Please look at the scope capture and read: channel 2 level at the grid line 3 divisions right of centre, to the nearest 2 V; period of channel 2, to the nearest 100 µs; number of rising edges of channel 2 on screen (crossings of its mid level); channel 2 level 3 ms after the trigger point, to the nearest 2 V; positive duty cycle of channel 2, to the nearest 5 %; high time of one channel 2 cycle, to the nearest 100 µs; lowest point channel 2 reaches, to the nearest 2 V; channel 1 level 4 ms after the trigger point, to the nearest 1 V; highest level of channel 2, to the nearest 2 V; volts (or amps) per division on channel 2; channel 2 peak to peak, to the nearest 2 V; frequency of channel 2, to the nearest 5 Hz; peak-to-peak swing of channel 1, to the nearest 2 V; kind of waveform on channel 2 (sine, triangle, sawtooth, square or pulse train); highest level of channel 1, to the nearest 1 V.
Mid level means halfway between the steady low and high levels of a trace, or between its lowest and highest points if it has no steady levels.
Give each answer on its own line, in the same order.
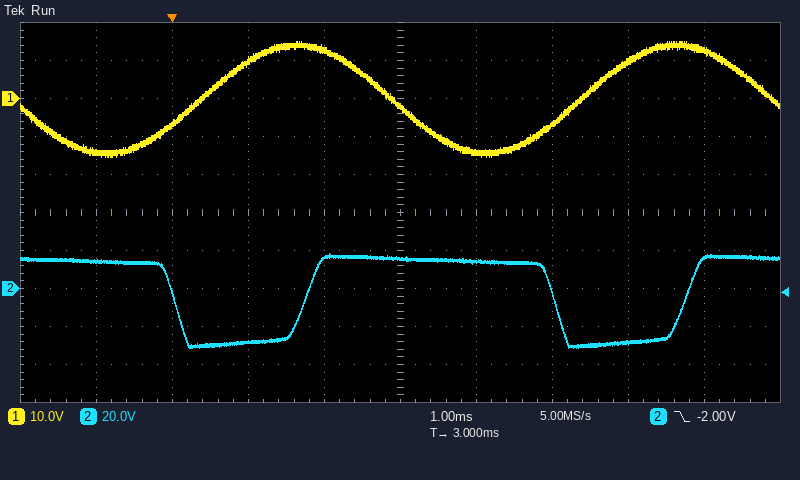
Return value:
-28 V
5.0 ms
2
16 V
65 %
3.3 ms
-32 V
-14 V
18 V
20 V
50 V
200 Hz
30 V
pulse train
15 V
